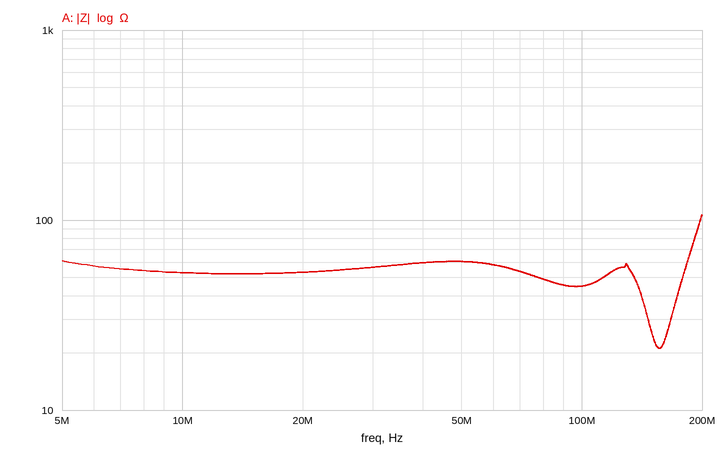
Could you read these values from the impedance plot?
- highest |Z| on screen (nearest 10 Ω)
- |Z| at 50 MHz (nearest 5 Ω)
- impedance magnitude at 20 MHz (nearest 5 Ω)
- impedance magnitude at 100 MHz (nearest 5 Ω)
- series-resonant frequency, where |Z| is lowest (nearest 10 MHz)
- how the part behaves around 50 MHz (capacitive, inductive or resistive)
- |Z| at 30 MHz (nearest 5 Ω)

110 Ω
60 Ω
55 Ω
45 Ω
160 MHz
resistive
55 Ω
